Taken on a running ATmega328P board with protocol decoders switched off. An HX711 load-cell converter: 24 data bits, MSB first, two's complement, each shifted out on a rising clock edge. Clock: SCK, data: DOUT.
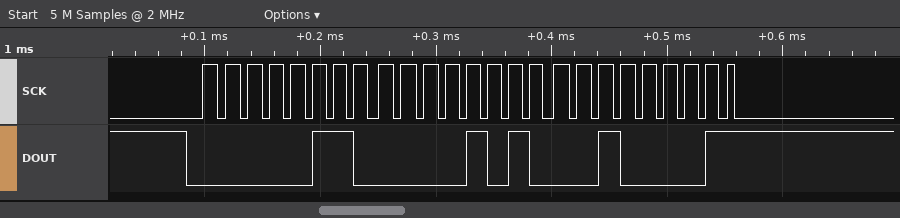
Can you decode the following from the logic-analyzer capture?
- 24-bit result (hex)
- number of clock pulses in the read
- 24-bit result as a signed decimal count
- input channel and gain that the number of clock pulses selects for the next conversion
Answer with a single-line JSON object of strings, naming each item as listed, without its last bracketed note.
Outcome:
{"24-bit result": "0x060A21", "number of clock pulses in the read": "25", "24-bit result as a signed decimal count": "395809", "input channel and gain that the number of clock pulses selects for the next conversion": "channel A, gain 128"}
